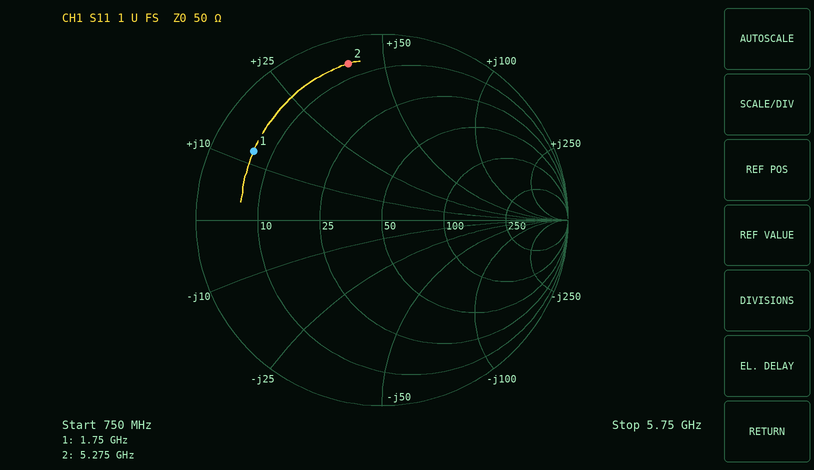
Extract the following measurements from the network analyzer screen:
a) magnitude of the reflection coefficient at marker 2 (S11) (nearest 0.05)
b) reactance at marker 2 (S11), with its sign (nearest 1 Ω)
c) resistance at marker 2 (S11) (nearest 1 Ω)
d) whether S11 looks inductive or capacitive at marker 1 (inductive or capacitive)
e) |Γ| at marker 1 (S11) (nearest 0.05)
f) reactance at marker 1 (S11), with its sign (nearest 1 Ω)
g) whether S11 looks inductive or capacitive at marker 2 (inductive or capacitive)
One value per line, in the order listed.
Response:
0.85
+40 Ω
6 Ω
inductive
0.80
+12 Ω
inductive
